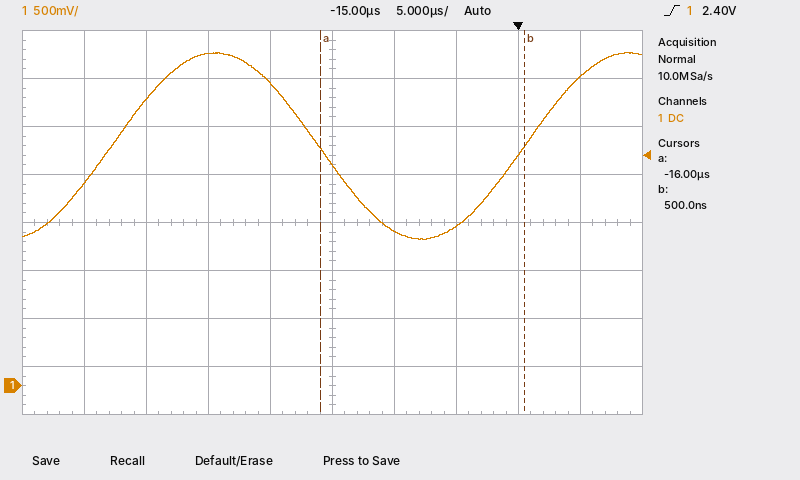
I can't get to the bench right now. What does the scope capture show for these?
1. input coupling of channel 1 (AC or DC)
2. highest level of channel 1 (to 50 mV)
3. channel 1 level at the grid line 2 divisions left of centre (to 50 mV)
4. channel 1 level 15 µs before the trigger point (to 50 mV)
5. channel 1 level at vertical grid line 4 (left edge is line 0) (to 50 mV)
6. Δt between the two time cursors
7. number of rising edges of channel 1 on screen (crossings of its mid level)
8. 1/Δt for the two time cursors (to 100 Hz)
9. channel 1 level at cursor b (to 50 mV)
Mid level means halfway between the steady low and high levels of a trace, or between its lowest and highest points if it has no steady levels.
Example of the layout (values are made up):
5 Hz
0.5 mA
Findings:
DC
3.45 V
3.45 V
2.30 V
3.15 V
16.5 µs
2
60.6 kHz
2.50 V
